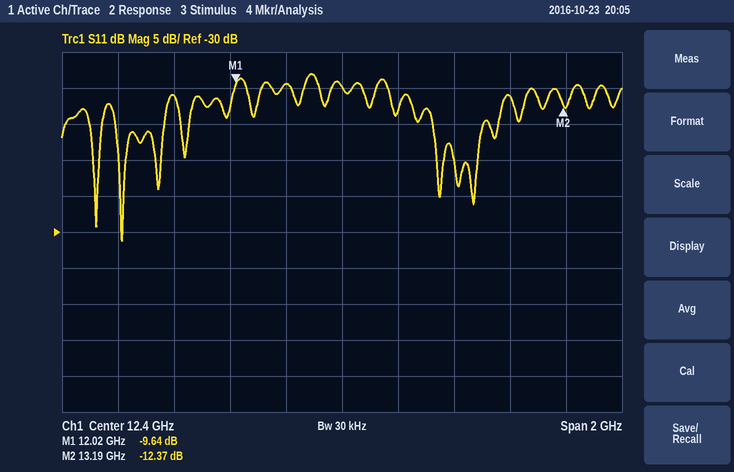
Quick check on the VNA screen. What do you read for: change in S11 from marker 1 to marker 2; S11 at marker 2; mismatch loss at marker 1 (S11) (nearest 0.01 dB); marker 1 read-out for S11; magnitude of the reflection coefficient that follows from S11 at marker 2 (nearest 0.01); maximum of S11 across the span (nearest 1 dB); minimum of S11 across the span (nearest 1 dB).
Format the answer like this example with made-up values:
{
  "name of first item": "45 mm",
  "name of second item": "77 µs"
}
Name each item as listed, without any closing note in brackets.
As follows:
{
  "change in S11 from marker 1 to marker 2": "-2.73 dB",
  "S11 at marker 2": "-12.37 dB",
  "mismatch loss at marker 1 (S11)": "0.50 dB",
  "marker 1 read-out for S11": "-9.64 dB",
  "magnitude of the reflection coefficient that follows from S11 at marker 2": "0.24",
  "maximum of S11 across the span": "-8 dB",
  "minimum of S11 across the span": "-31 dB"
}
